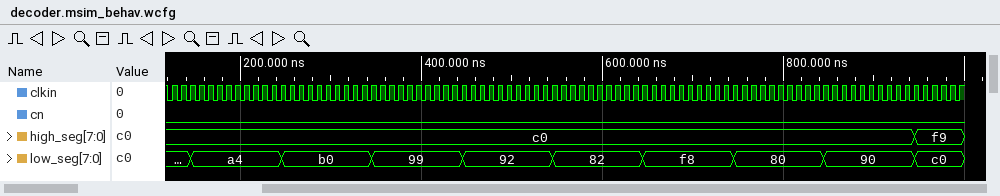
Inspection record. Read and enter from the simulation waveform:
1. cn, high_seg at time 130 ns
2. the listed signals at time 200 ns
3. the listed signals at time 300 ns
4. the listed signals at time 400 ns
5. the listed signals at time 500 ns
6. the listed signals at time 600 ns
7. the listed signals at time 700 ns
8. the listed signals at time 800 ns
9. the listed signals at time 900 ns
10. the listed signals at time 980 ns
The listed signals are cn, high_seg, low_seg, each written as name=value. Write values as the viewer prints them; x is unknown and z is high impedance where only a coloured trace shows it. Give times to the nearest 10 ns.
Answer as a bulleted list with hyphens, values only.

- cn=0, high_seg=c0
- cn=0, high_seg=c0, low_seg=a4
- cn=0, high_seg=c0, low_seg=b0
- cn=0, high_seg=c0, low_seg=99
- cn=0, high_seg=c0, low_seg=92
- cn=0, high_seg=c0, low_seg=82
- cn=0, high_seg=c0, low_seg=f8
- cn=0, high_seg=c0, low_seg=80
- cn=0, high_seg=c0, low_seg=90
- cn=0, high_seg=f9, low_seg=c0
